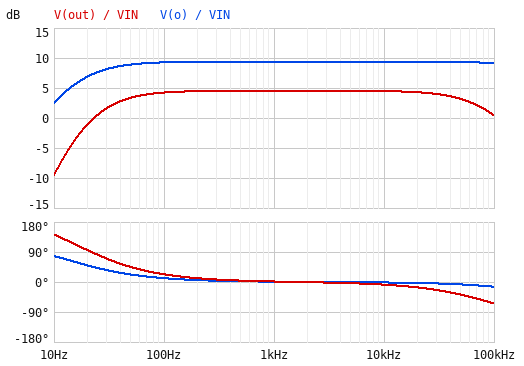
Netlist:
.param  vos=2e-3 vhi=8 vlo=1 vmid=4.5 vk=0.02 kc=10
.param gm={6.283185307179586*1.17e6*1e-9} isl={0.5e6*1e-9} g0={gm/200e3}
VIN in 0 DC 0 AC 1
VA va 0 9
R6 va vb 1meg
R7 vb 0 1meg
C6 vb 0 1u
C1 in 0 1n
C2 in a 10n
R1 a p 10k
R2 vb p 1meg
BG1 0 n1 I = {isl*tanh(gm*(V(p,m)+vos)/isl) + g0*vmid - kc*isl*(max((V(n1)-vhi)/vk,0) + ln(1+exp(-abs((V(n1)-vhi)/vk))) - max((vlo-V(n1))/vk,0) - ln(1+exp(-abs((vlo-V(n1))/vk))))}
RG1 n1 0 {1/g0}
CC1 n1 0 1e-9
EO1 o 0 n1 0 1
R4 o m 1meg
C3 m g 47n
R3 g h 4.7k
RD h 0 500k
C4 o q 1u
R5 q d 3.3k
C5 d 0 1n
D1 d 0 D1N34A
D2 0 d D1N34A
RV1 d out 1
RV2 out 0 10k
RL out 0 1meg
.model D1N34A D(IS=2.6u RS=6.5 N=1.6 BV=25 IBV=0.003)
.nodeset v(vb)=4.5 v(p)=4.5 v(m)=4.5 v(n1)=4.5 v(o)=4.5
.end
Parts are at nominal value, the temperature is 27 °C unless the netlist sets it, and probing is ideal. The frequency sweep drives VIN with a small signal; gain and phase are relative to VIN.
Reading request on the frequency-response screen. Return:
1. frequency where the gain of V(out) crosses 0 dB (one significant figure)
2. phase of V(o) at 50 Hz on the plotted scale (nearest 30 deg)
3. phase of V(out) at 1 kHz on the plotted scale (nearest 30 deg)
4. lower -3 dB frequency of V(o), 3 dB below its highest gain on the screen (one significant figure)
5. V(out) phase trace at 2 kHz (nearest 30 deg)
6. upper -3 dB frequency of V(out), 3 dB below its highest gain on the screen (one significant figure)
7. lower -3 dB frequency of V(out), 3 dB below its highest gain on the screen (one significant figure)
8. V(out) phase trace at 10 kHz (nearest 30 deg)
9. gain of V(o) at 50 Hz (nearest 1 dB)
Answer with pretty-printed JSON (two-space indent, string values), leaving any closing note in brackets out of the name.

{
  "frequency where the gain of V(out) crosses 0 dB": "20 Hz",
  "phase of V(o) at 50 Hz on the plotted scale": "30 deg",
  "phase of V(out) at 1 kHz on the plotted scale": "0 deg",
  "lower -3 dB frequency of V(o), 3 dB below its highest gain on the screen": "20 Hz",
  "V(out) phase trace at 2 kHz": "0 deg",
  "upper -3 dB frequency of V(out), 3 dB below its highest gain on the screen": "80 kHz",
  "lower -3 dB frequency of V(out), 3 dB below its highest gain on the screen": "30 Hz",
  "V(out) phase trace at 10 kHz": "0 deg",
  "gain of V(o) at 50 Hz": "9 dB"
}
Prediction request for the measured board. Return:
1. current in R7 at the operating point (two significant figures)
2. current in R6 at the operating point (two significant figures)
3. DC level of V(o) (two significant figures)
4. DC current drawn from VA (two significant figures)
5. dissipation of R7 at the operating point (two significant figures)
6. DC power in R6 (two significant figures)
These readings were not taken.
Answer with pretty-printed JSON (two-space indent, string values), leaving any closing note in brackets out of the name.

{
  "current in R7 at the operating point": "4.5 µA",
  "current in R6 at the operating point": "4.5 µA",
  "DC level of V(o)": "4.5 V",
  "DC current drawn from VA": "4.5 µA",
  "dissipation of R7 at the operating point": "20 µW",
  "DC power in R6": "20 µW"
}
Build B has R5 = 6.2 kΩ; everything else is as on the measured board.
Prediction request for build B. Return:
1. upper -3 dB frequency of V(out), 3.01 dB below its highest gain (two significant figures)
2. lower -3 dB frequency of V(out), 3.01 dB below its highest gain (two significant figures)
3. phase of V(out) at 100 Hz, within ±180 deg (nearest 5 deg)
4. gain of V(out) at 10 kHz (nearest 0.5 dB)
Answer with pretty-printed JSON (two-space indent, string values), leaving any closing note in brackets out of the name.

{
  "upper -3 dB frequency of V(out), 3.01 dB below its highest gain": "60 kHz",
  "lower -3 dB frequency of V(out), 3.01 dB below its highest gain": "25 Hz",
  "phase of V(out) at 100 Hz, within ±180 deg": "20 deg",
  "gain of V(out) at 10 kHz": "1.5 dB"
}
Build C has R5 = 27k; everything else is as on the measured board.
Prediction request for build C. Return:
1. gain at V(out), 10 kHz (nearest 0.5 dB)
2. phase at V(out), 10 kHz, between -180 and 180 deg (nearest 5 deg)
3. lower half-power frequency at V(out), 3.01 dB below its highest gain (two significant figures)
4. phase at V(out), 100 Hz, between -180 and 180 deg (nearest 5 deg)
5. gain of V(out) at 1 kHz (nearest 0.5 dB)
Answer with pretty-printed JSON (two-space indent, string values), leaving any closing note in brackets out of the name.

{
  "gain at V(out), 10 kHz": "-8.0 dB",
  "phase at V(out), 10 kHz, between -180 and 180 deg": "-15 deg",
  "lower half-power frequency at V(out), 3.01 dB below its highest gain": "19 Hz",
  "phase at V(out), 100 Hz, between -180 and 180 deg": "15 deg",
  "gain of V(out) at 1 kHz": "-7.5 dB"
}
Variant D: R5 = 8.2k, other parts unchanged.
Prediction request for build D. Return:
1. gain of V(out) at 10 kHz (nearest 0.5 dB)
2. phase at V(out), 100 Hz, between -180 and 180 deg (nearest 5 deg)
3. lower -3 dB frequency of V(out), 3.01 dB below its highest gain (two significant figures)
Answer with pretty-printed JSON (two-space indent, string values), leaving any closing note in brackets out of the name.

{
  "gain of V(out) at 10 kHz": "0 dB",
  "phase at V(out), 100 Hz, between -180 and 180 deg": "20 deg",
  "lower -3 dB frequency of V(out), 3.01 dB below its highest gain": "24 Hz"
}
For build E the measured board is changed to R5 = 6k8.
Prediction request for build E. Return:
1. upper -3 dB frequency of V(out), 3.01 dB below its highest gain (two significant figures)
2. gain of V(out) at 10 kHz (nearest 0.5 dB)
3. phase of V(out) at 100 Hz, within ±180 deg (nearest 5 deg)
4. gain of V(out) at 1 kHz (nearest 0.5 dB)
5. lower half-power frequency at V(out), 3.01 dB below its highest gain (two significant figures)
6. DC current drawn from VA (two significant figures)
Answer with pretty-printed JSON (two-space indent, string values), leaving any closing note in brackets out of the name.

{
  "upper -3 dB frequency of V(out), 3.01 dB below its highest gain": "58 kHz",
  "gain of V(out) at 10 kHz": "1.0 dB",
  "phase of V(out) at 100 Hz, within ±180 deg": "20 deg",
  "gain of V(out) at 1 kHz": "1.5 dB",
  "lower half-power frequency at V(out), 3.01 dB below its highest gain": "25 Hz",
  "DC current drawn from VA": "4.5 µA"
}
